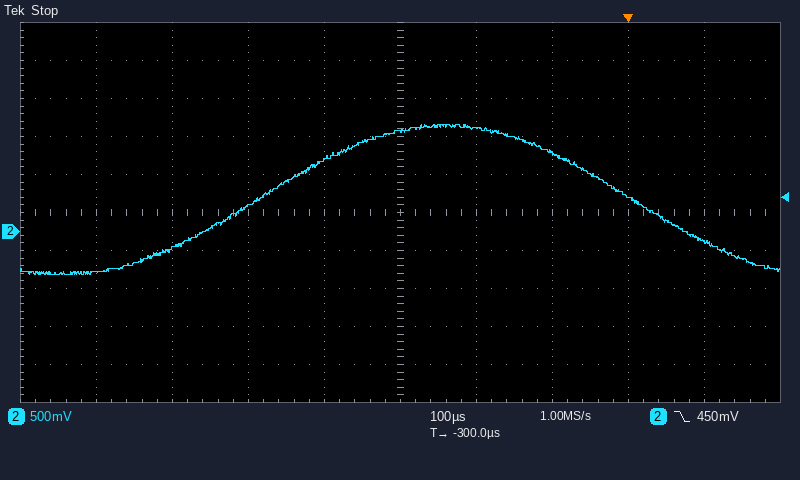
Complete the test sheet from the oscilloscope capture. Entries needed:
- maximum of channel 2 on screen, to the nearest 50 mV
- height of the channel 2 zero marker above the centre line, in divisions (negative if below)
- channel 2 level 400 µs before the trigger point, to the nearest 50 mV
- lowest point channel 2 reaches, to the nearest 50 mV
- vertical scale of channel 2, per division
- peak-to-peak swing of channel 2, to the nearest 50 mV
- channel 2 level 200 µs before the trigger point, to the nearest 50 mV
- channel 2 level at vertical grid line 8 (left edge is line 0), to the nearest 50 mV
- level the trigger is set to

1.40 V
-0.5 div
950 mV
-550 mV
500 mV
1.95 V
1.35 V
450 mV
450 mV
